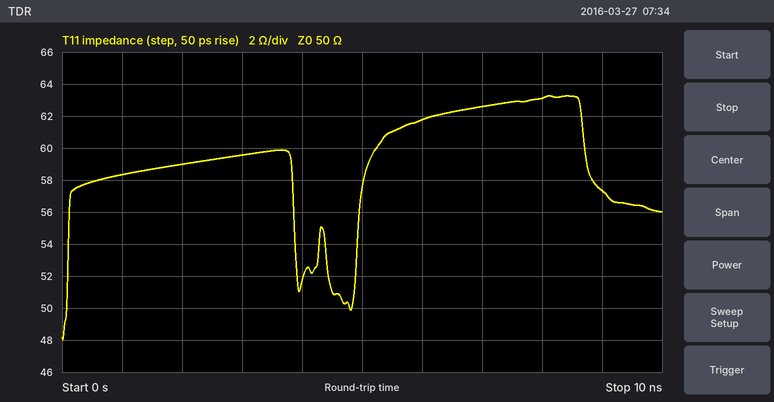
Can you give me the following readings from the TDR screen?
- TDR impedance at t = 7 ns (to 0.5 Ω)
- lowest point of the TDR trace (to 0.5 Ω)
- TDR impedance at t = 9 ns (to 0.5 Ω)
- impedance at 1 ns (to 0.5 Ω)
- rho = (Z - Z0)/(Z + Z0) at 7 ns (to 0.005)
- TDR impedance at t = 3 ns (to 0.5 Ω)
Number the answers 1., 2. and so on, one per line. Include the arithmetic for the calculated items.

1. 62.5 Ω
2. 48.0 Ω
3. 57.5 Ω
4. 58.5 Ω
5. (62.5 − 50)/(62.5 + 50) ≈ +0.111, so +0.110 to the nearest 0.005
6. 59.5 Ω
